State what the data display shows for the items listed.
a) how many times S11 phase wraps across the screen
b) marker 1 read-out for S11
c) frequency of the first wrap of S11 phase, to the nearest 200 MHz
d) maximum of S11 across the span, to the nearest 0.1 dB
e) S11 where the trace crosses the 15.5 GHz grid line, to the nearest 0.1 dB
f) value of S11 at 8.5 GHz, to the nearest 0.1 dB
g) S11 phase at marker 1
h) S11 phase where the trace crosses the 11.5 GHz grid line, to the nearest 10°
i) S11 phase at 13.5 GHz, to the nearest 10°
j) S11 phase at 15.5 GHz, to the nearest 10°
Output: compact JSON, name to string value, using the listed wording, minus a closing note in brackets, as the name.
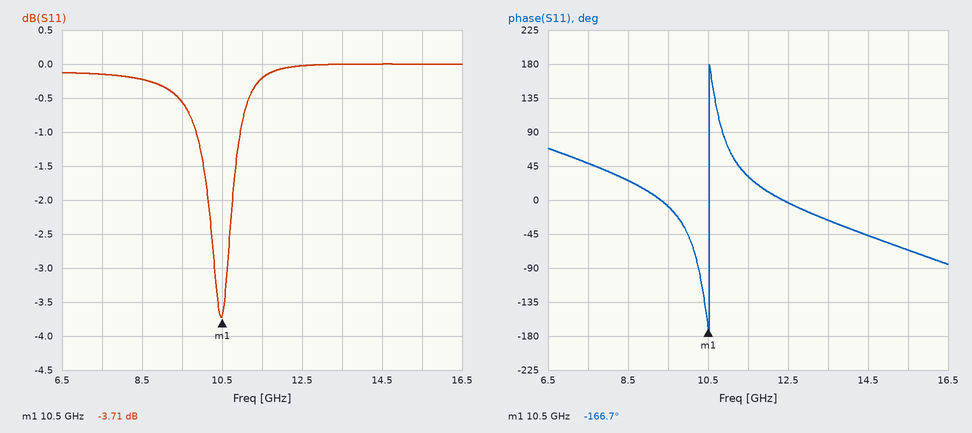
{"how many times S11 phase wraps across the screen": "1", "marker 1 read-out for S11": "-3.71 dB", "frequency of the first wrap of S11 phase, to the nearest 200 MHz": "10.6 GHz", "maximum of S11 across the span, to the nearest 0.1 dB": "0.0 dB", "S11 where the trace crosses the 15.5 GHz grid line, to the nearest 0.1 dB": "0.0 dB", "value of S11 at 8.5 GHz, to the nearest 0.1 dB": "-0.2 dB", "S11 phase at marker 1": "-166.7°", "S11 phase where the trace crosses the 11.5 GHz grid line, to the nearest 10°": "30°", "S11 phase at 13.5 GHz, to the nearest 10°": "-30°", "S11 phase at 15.5 GHz, to the nearest 10°": "-70°"}
